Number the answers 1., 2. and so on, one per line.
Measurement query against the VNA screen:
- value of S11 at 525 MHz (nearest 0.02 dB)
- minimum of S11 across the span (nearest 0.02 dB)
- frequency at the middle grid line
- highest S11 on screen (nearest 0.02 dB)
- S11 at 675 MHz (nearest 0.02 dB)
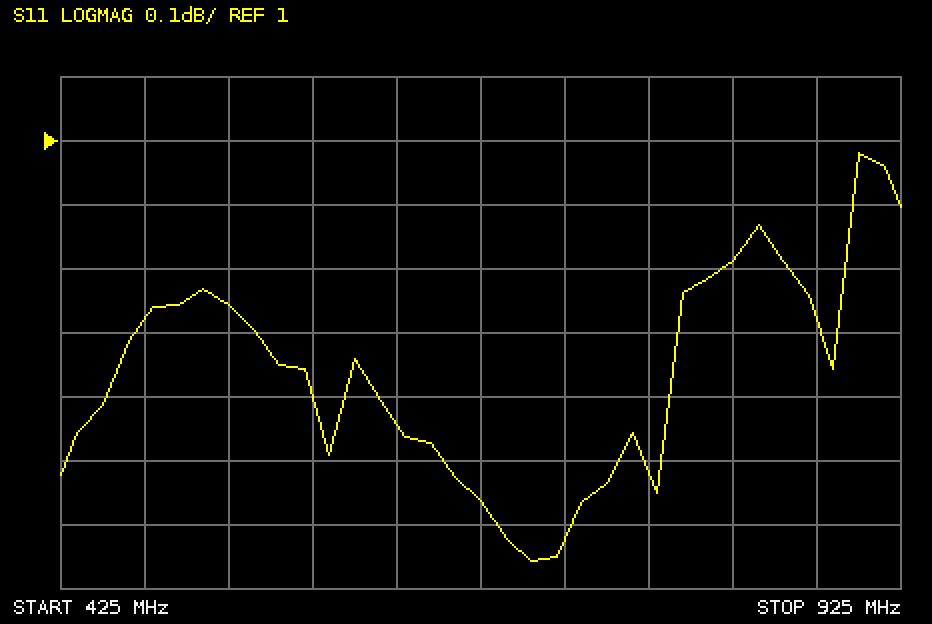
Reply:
1. 0.74 dB
2. 0.34 dB
3. 675 MHz
4. 0.98 dB
5. 0.44 dB
